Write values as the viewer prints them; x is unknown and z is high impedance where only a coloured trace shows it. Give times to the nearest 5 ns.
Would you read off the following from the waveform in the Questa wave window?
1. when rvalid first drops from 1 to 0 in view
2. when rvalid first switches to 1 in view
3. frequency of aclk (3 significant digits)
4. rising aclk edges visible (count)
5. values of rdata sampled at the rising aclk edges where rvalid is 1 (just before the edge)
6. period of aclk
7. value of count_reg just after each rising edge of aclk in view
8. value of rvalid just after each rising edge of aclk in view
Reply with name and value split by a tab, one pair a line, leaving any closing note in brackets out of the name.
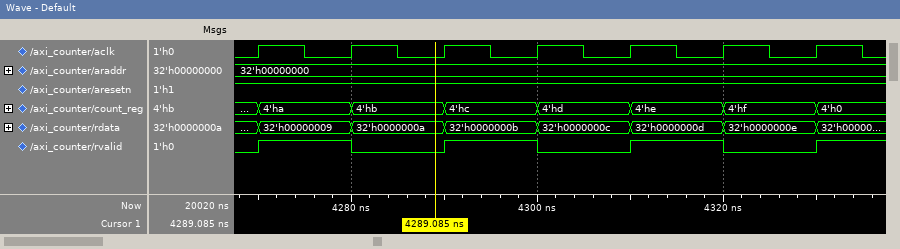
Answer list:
when rvalid first drops from 1 to 0 in view	4280 ns
when rvalid first switches to 1 in view	4270 ns
frequency of aclk	100 MHz
rising aclk edges visible	7
values of rdata sampled at the rising aclk edges where rvalid is 1	32'h00000009, 32'h0000000b, 32'h0000000d
period of aclk	10 ns
value of count_reg just after each rising edge of aclk in view	4'ha, 4'hb, 4'hc, 4'hd, 4'he, 4'hf, 4'h0
value of rvalid just after each rising edge of aclk in view	1 0 1 0 1 0 1
